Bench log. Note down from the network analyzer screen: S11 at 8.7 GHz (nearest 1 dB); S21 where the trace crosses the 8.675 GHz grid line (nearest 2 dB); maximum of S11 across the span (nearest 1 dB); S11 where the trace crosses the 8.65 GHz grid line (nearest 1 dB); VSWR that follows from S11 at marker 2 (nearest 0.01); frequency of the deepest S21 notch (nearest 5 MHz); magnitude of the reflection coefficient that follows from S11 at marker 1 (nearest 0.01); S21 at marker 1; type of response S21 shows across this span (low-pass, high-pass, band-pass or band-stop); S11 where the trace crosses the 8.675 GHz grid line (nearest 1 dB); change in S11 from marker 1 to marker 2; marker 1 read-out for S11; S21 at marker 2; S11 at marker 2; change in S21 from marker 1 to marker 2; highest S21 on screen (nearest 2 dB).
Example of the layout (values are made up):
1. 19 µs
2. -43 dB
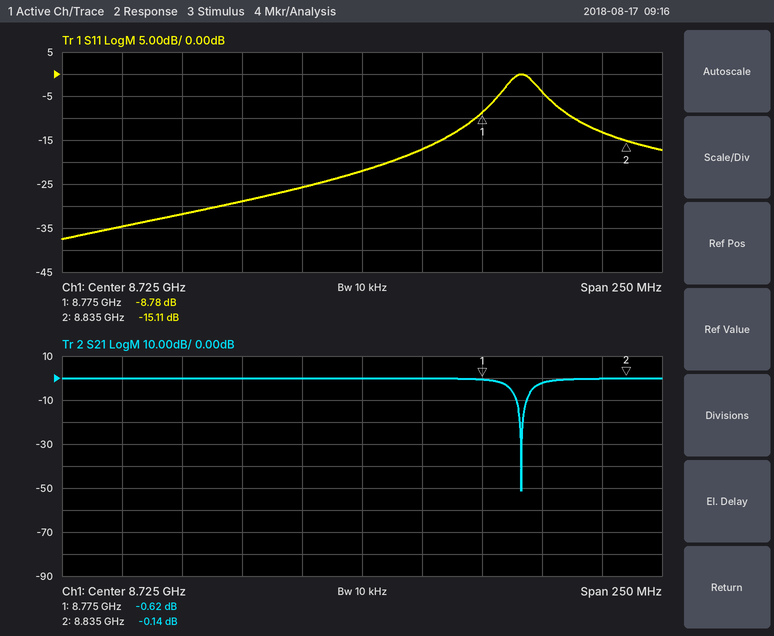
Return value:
1. -26 dB
2. 0 dB
3. 0 dB
4. -32 dB
5. 1.43
6. 8.790 GHz
7. 0.36
8. -0.62 dB
9. band-stop
10. -29 dB
11. -6.33 dB
12. -8.78 dB
13. -0.14 dB
14. -15.11 dB
15. 0.48 dB
16. 0 dB
